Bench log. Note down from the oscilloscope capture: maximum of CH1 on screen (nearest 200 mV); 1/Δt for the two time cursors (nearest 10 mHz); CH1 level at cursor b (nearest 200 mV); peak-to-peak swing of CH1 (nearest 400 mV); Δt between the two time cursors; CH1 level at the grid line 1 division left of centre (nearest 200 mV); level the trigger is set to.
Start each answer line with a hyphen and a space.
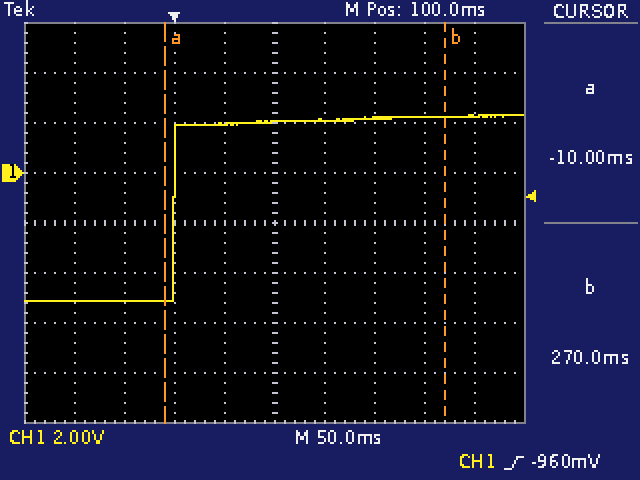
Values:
- 2.4 V
- 3.57 Hz
- 2.2 V
- 7.6 V
- 280 ms
- 2.0 V
- -960 mV
